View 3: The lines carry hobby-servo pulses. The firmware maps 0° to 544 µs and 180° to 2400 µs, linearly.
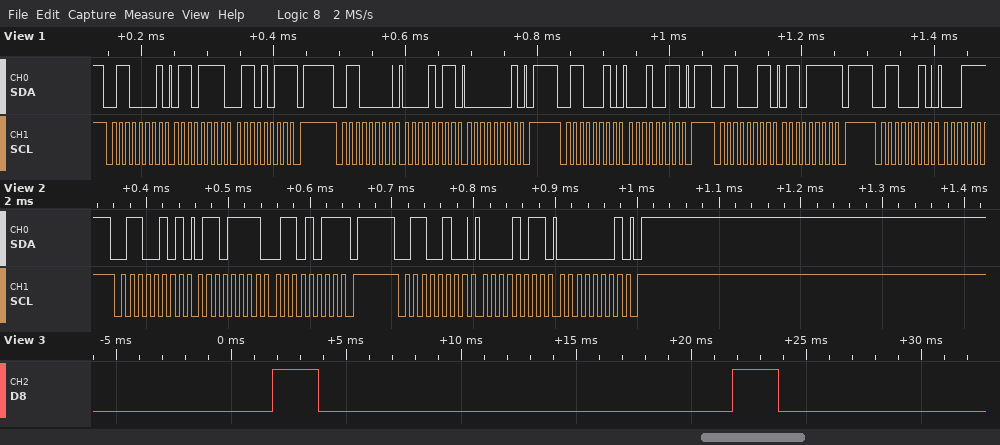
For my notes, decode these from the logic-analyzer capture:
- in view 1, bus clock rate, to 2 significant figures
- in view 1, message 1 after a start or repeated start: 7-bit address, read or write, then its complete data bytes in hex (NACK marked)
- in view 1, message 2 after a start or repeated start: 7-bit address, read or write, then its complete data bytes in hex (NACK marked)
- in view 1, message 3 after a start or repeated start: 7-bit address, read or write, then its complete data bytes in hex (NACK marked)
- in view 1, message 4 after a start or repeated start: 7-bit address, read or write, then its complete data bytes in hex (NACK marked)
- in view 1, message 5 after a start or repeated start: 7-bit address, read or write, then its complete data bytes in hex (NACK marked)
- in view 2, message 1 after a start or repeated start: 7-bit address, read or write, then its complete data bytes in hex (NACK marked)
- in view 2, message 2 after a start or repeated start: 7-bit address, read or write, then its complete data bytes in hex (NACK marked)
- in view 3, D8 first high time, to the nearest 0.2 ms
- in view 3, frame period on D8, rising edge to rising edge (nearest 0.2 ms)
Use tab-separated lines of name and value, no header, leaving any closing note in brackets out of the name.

in view 1, bus clock rate, to 2 significant figures	100 kHz
in view 1, message 1 after a start or repeated start: 7-bit address, read or write, then its complete data bytes in hex	0x30 read: 6F 6B NACK
in view 1, message 2 after a start or repeated start: 7-bit address, read or write, then its complete data bytes in hex	0x30 write: 0B 01
in view 1, message 3 after a start or repeated start: 7-bit address, read or write, then its complete data bytes in hex	0x31 write: 13
in view 1, message 4 after a start or repeated start: 7-bit address, read or write, then its complete data bytes in hex	0x31 read: 6F NACK
in view 1, message 5 after a start or repeated start: 7-bit address, read or write, then its complete data bytes in hex	0x31 write
in view 2, message 1 after a start or repeated start: 7-bit address, read or write, then its complete data bytes in hex	0x32 read: 6F 6B NACK
in view 2, message 2 after a start or repeated start: 7-bit address, read or write, then its complete data bytes in hex	0x32 write: 0B 01
in view 3, D8 first high time, to the nearest 0.2 ms	2.0 ms
in view 3, frame period on D8, rising edge to rising edge	20.0 ms
